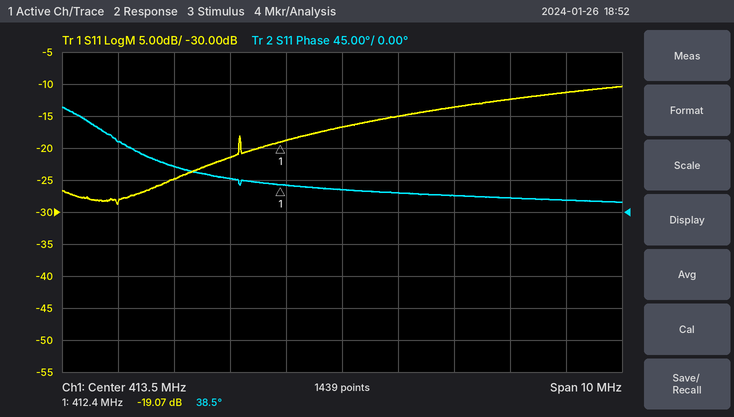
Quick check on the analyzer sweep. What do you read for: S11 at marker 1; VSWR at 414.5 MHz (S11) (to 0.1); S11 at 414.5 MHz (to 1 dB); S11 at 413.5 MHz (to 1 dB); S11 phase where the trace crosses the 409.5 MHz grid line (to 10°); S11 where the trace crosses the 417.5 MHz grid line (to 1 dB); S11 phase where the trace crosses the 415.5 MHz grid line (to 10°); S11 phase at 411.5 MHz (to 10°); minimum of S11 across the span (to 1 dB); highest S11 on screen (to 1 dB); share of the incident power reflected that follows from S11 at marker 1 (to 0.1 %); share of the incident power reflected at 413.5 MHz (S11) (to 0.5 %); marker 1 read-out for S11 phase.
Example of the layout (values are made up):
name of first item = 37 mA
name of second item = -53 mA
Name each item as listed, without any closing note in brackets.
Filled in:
S11 at marker 1 = -19.07 dB
VSWR at 414.5 MHz (S11) = 1.4
S11 at 414.5 MHz = -15 dB
S11 at 413.5 MHz = -17 dB
S11 phase where the trace crosses the 409.5 MHz grid line = 100°
S11 where the trace crosses the 417.5 MHz grid line = -11 dB
S11 phase where the trace crosses the 415.5 MHz grid line = 20°
S11 phase at 411.5 MHz = 50°
minimum of S11 across the span = -29 dB
highest S11 on screen = -10 dB
share of the incident power reflected that follows from S11 at marker 1 = 1.2 %
share of the incident power reflected at 413.5 MHz (S11) = 2.0 %
marker 1 read-out for S11 phase = 38.5°
